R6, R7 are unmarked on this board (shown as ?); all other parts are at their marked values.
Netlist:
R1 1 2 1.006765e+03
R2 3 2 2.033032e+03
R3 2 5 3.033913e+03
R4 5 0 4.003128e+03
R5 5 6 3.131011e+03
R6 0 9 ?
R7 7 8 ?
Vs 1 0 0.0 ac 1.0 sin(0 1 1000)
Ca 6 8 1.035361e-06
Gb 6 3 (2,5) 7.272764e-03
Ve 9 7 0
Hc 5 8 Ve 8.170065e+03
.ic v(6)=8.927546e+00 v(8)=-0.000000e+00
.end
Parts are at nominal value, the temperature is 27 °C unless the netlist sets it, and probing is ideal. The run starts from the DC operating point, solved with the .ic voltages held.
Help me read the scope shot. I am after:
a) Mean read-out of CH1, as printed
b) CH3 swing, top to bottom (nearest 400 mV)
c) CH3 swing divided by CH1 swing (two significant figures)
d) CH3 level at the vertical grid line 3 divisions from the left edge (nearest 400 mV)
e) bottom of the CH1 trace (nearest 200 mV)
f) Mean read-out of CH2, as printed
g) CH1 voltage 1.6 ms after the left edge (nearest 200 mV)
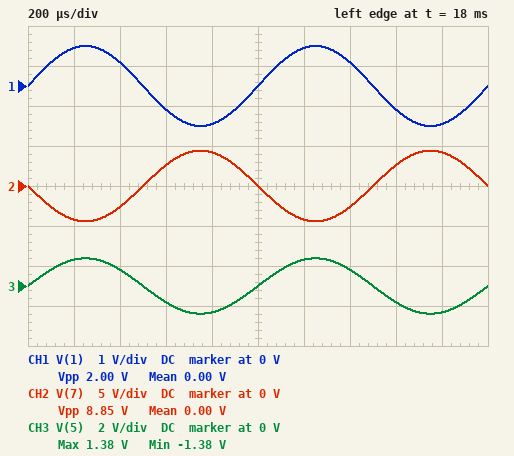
0.00 V
2.8 V
1.4
-800 mV
-1.0 V
0.00 V
-600 mV
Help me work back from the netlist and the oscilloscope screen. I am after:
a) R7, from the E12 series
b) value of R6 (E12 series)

820 Ω
5.6 kΩ
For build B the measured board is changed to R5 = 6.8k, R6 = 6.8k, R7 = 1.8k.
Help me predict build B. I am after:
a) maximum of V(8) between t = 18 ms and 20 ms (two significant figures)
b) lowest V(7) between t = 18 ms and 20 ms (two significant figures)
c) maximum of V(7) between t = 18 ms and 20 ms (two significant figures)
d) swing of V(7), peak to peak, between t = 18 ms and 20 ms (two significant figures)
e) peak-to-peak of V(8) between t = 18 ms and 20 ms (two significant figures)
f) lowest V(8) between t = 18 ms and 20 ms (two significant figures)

6.2 V
-4.9 V
4.9 V
9.8 V
12 V
-6.2 V
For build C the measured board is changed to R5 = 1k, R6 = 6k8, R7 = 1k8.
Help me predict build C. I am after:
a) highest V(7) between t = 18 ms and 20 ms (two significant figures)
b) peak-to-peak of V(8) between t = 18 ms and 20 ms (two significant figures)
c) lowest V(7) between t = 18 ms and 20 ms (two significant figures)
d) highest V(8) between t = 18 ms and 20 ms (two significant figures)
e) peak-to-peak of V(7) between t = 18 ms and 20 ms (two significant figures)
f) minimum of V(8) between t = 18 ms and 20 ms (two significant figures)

4.9 V
12 V
-4.9 V
6.2 V
9.8 V
-6.2 V
